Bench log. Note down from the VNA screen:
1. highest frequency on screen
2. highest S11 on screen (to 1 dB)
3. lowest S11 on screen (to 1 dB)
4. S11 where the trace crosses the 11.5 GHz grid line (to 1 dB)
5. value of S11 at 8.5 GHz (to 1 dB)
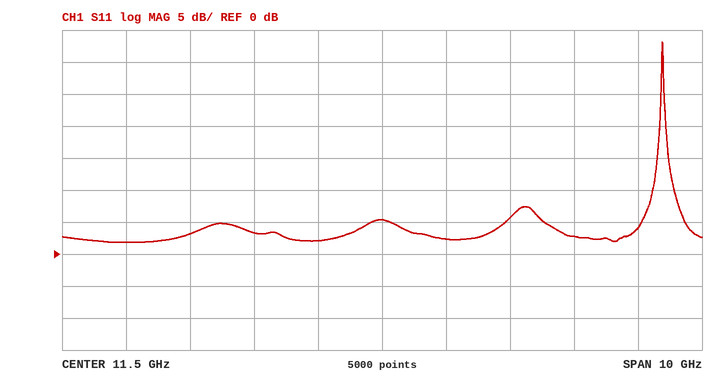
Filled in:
16.5 GHz
33 dB
2 dB
5 dB
3 dB
